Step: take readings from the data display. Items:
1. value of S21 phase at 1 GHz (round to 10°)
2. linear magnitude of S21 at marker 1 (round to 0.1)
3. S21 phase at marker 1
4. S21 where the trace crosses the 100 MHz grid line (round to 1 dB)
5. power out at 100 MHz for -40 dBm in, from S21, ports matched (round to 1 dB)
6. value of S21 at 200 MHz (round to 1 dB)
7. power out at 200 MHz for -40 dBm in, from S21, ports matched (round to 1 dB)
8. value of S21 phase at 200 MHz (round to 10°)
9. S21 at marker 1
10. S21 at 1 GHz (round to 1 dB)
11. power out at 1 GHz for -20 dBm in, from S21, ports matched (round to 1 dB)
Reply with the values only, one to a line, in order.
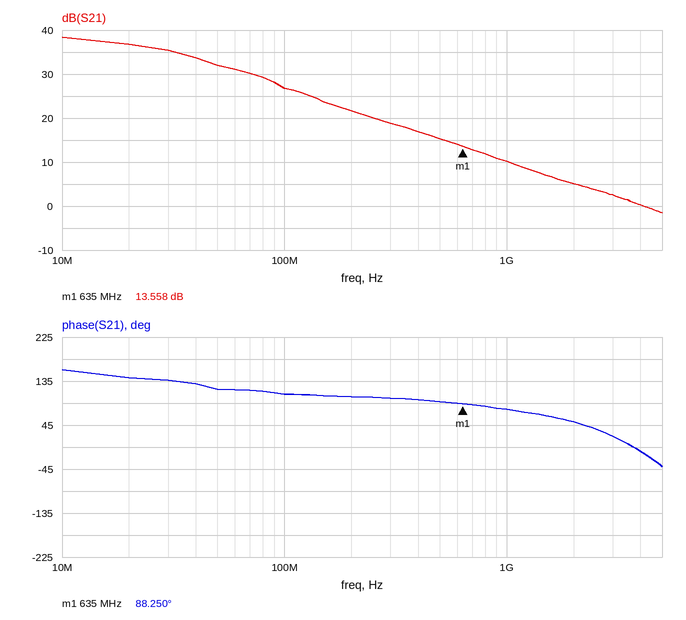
80°
4.8
88.250°
27 dB
-13 dBm
22 dB
-18 dBm
100°
13.558 dB
10 dB
-10 dBm
